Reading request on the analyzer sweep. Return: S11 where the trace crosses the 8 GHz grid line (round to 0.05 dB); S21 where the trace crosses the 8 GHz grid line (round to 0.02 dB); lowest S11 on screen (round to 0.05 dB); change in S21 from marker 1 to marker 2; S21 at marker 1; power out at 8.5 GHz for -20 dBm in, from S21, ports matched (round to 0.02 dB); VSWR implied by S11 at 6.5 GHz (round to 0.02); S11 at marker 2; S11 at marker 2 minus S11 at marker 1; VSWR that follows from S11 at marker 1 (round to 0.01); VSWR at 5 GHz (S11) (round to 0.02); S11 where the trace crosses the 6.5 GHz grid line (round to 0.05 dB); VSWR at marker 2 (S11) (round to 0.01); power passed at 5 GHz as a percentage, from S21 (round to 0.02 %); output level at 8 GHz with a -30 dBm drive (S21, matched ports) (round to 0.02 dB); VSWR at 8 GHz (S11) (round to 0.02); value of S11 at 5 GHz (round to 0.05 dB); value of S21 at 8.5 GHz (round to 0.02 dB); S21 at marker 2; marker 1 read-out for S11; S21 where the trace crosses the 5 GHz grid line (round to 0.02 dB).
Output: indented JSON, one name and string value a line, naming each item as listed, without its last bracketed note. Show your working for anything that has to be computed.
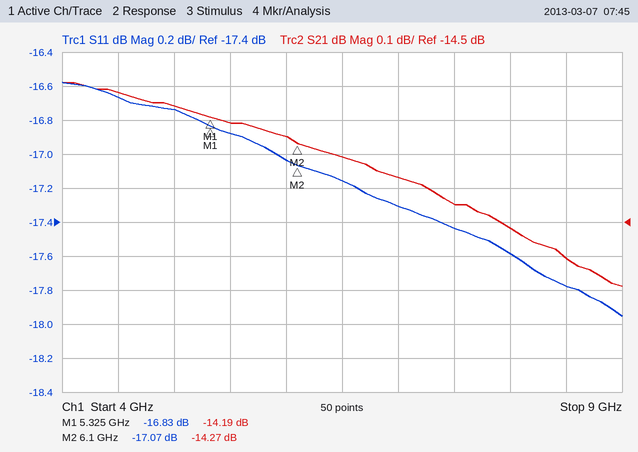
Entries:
{
  "S11 where the trace crosses the 8 GHz grid line": "-17.60 dB",
  "S21 where the trace crosses the 8 GHz grid line": "-14.52 dB",
  "lowest S11 on screen": "-17.95 dB",
  "change in S21 from marker 1 to marker 2": "-14.27 − (-14.19) = -0.08 dB",
  "S21 at marker 1": "-14.19 dB",
  "power out at 8.5 GHz for -20 dBm in, from S21, ports matched": "-20 dBm + (-14.60 dB) = -34.60 dBm",
  "VSWR implied by S11 at 6.5 GHz": "|Γ| = 10^(-17.15/20) = 0.1388; VSWR = (1 + 0.1388)/(1 − 0.1388) ≈ 1.32",
  "S11 at marker 2": "-17.07 dB",
  "S11 at marker 2 minus S11 at marker 1": "-17.07 − (-16.83) = -0.24 dB",
  "VSWR that follows from S11 at marker 1": "(1 + 0.1440)/(1 − 0.1440) ≈ 1.34",
  "VSWR at 5 GHz (S11)": "|Γ| = 10^(-16.75/20) = 0.1454; VSWR = (1 + 0.1454)/(1 − 0.1454) ≈ 1.34",
  "S11 where the trace crosses the 6.5 GHz grid line": "-17.15 dB",
  "VSWR at marker 2 (S11)": "(1 + 0.1401)/(1 − 0.1401) ≈ 1.33",
  "power passed at 5 GHz as a percentage, from S21": "10^(-14.16/10) ≈ 3.84 %",
  "output level at 8 GHz with a -30 dBm drive (S21, matched ports)": "-30 dBm + (-14.52 dB) = -44.52 dBm",
  "VSWR at 8 GHz (S11)": "|Γ| = 10^(-17.6/20) = 0.1318; VSWR = (1 + 0.1318)/(1 − 0.1318) ≈ 1.30",
  "value of S11 at 5 GHz": "-16.75 dB",
  "value of S21 at 8.5 GHz": "-14.60 dB",
  "S21 at marker 2": "-14.27 dB",
  "marker 1 read-out for S11": "-16.83 dB",
  "S21 where the trace crosses the 5 GHz grid line": "-14.16 dB"
}
